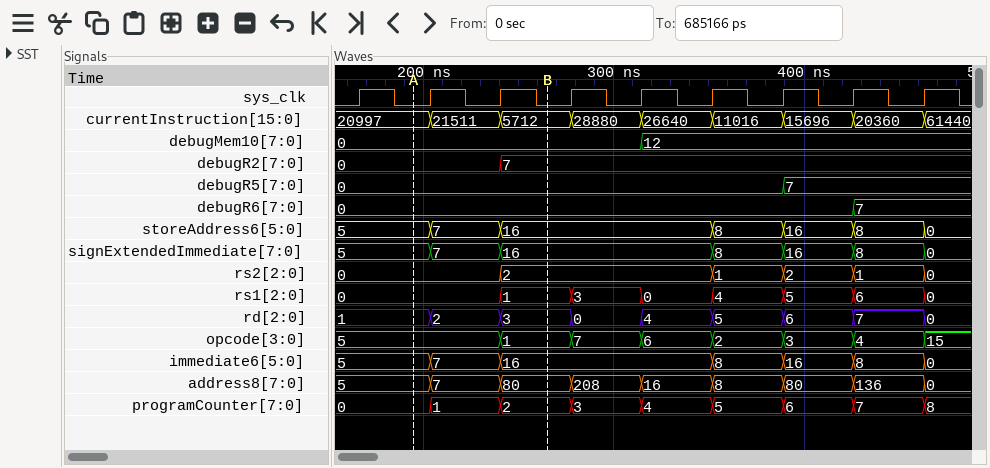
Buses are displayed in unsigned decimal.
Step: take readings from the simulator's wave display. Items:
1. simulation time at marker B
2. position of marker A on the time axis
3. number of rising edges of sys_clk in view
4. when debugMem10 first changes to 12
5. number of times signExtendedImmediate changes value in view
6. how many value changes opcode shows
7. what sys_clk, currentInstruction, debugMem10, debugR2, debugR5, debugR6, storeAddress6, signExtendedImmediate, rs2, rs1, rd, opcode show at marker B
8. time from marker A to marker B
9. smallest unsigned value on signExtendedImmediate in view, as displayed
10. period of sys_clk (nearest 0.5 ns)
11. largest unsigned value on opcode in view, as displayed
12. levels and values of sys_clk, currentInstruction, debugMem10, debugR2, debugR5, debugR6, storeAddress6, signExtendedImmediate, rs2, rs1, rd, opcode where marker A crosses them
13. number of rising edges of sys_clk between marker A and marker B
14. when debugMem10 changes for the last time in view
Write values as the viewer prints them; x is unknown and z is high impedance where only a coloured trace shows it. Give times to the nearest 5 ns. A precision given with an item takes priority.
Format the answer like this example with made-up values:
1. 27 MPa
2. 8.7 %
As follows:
1. 265 ns
2. 195 ns
3. 9
4. 315 ns
5. 6
6. 7
7. sys_clk=0, currentInstruction=5712, debugMem10=0, debugR2=7, debugR5=0, debugR6=0, storeAddress6=16, signExtendedImmediate=16, rs2=2, rs1=1, rd=3, opcode=1
8. 70 ns
9. 0
10. 37 ns
11. 15
12. sys_clk=0, currentInstruction=20997, debugMem10=0, debugR2=0, debugR5=0, debugR6=0, storeAddress6=5, signExtendedImmediate=5, rs2=0, rs1=0, rd=1, opcode=5
13. 2
14. 315 ns
